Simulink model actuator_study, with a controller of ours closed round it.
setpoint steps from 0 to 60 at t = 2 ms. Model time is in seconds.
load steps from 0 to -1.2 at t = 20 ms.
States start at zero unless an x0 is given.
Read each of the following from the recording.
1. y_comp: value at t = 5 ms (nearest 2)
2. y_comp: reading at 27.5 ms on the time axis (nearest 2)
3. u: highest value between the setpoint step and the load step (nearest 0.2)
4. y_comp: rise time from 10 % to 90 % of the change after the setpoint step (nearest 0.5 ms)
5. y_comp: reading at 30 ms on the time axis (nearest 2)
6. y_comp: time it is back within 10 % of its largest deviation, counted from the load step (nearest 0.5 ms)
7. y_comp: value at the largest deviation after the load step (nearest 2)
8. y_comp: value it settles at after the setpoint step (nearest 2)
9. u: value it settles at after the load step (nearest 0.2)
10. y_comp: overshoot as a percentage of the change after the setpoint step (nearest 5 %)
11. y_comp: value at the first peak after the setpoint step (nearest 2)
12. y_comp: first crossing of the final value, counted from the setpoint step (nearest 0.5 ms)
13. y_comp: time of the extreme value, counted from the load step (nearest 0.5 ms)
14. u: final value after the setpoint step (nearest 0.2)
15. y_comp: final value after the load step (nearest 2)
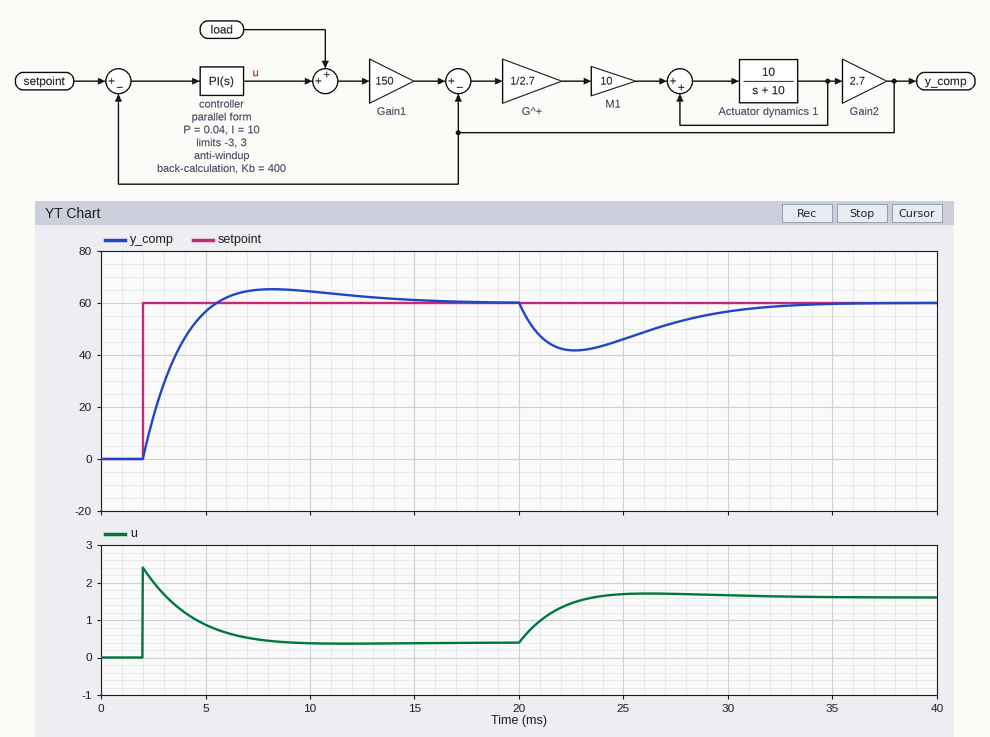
56
52
2.4
2.5 ms
56
11.5 ms
42
60
1.6
10 %
66
3.5 ms
2.5 ms
0.4
60
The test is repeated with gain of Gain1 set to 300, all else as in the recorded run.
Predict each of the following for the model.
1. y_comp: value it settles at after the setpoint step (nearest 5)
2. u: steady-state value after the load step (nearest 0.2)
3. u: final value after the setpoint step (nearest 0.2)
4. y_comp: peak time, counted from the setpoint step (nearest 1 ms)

60
1.4
0.2
4 ms
